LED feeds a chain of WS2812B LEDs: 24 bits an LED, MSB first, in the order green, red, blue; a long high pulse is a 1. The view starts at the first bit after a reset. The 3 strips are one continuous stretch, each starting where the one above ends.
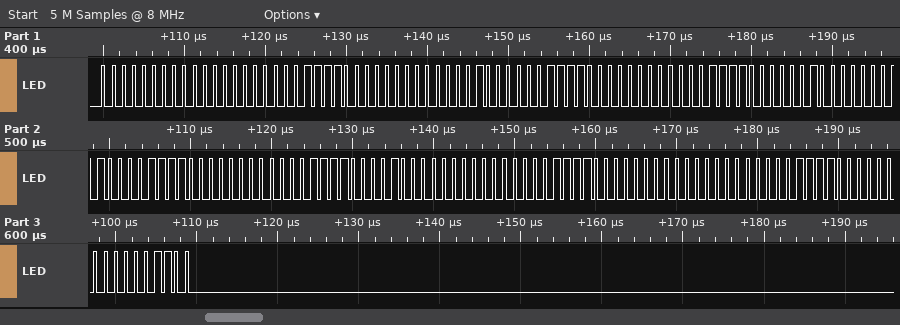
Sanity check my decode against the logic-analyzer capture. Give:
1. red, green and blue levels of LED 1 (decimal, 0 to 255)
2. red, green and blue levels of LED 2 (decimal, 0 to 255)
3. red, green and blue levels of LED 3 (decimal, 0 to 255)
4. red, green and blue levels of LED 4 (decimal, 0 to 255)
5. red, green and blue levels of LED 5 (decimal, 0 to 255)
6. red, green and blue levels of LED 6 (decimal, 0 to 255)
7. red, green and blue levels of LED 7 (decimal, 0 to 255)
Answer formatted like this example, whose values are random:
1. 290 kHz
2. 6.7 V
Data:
1. 0, 0, 15
2. 4, 0, 15
3. 15, 0, 2
4. 15, 1, 0
5. 8, 15, 0
6. 0, 15, 0
7. 0, 15, 12
